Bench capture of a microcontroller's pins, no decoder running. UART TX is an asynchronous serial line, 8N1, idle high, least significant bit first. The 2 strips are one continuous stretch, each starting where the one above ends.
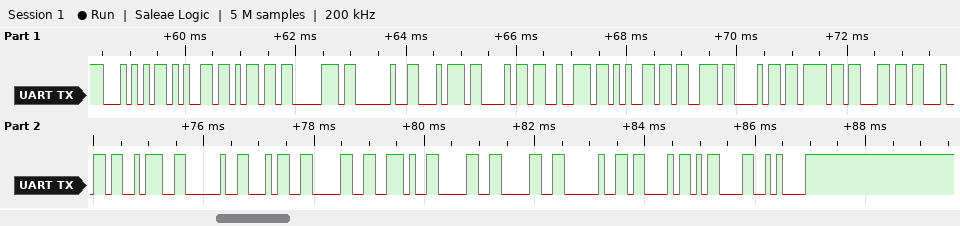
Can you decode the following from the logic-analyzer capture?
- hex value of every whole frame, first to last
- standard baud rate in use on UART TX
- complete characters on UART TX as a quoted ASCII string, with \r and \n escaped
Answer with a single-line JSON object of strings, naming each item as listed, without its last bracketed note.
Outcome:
{"hex value of every whole frame, first to last": "54 65 6D 70 20 74 68 72 65 73 68 6F 6C 64 3A 20 34 30 2E 30 30 20 43 0D 0A", "standard baud rate in use on UART TX": "9600 baud", "complete characters on UART TX as a quoted ASCII string, with \\r and \\n escaped": "\"Temp threshold: 40.00 C\\r\\n\""}
